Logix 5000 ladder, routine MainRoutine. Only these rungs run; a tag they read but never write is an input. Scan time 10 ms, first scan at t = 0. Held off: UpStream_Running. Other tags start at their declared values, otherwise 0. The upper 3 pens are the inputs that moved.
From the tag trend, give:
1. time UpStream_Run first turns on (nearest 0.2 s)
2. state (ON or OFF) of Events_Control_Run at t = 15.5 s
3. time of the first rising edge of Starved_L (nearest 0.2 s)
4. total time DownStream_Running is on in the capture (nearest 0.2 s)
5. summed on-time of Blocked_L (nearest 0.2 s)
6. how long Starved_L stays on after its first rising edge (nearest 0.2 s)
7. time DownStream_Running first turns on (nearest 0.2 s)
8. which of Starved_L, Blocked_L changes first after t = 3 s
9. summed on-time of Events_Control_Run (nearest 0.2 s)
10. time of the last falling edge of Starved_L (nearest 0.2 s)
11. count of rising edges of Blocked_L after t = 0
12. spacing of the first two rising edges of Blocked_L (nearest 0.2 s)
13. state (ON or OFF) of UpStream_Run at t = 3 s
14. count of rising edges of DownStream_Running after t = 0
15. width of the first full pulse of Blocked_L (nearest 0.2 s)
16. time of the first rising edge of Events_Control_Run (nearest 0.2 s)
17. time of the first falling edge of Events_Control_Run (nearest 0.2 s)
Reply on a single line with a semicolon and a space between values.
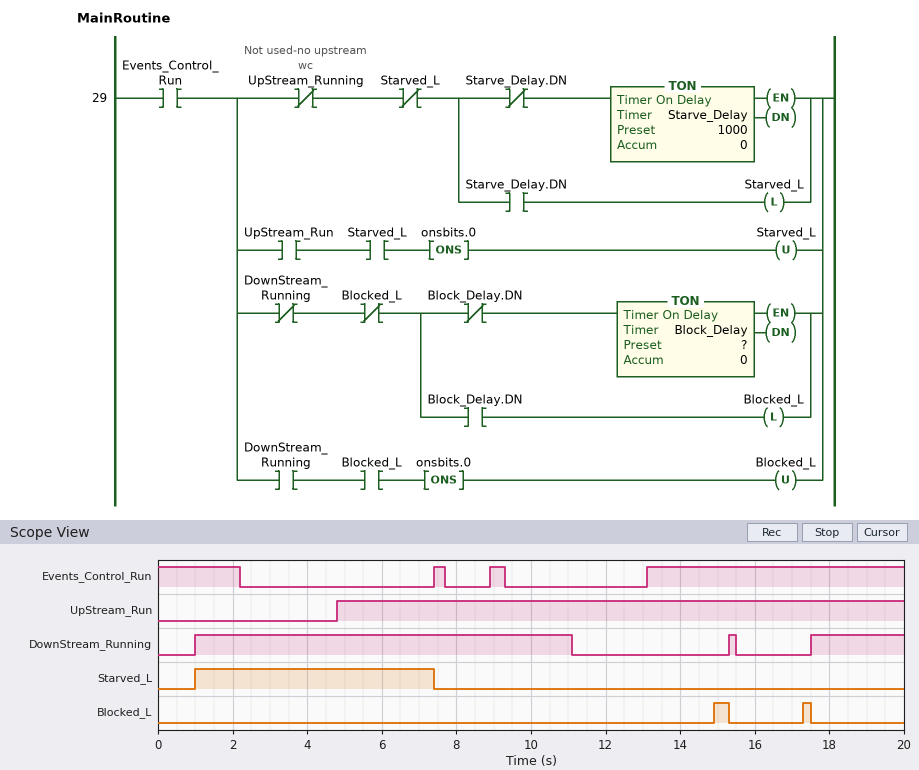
4.8 s; ON; 1.0 s; 12.8 s; 0.6 s; 6.4 s; 1.0 s; Starved_L; 9.8 s; 7.4 s; 2; 2.4 s; OFF; 3; 0.4 s; 7.4 s; 2.2 s
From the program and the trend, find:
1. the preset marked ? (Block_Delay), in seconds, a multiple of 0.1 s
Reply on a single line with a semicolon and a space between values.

1.8 s
